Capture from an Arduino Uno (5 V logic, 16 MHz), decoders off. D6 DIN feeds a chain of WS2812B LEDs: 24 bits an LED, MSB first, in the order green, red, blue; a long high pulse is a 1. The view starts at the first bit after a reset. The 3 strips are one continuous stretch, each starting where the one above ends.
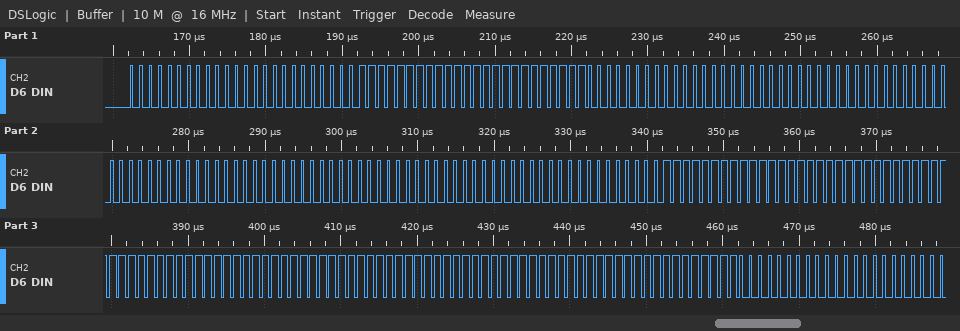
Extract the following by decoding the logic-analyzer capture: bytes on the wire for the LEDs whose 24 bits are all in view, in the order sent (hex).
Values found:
00 00 00 FF FF FF 00 00 00 00 00 00 00 00 00 00 00 00 FF FF FF FF FF FF FF FF FF FF FF FF
